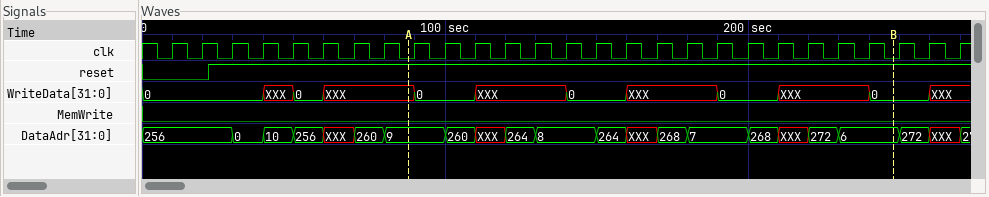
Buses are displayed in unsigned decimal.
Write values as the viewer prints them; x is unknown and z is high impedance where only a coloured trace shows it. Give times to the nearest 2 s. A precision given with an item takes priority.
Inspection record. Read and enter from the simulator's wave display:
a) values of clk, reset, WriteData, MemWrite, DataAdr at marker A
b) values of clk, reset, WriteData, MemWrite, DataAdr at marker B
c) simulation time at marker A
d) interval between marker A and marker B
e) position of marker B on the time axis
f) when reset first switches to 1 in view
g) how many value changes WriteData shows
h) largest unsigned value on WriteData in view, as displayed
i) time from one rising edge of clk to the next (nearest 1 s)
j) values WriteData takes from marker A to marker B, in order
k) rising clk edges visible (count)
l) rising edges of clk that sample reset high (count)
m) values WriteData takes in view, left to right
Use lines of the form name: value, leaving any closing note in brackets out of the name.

values of clk, reset, WriteData, MemWrite, DataAdr at marker A: clk=0, reset=1, WriteData=XXX, MemWrite=0, DataAdr=9
values of clk, reset, WriteData, MemWrite, DataAdr at marker B: clk=0, reset=1, WriteData=0, MemWrite=0, DataAdr=6
simulation time at marker A: 88 s
interval between marker A and marker B: 160 s
position of marker B on the time axis: 248 s
when reset first switches to 1 in view: 22 s
how many value changes WriteData shows: 11
largest unsigned value on WriteData in view, as displayed: 0
time from one rising edge of clk to the next: 10 s
values WriteData takes from marker A to marker B, in order: XXX, 0, XXX, 0, XXX, 0, XXX, 0
rising clk edges visible: 27
rising edges of clk that sample reset high: 25
values WriteData takes in view, left to right: 0, XXX, 0, XXX, 0, XXX, 0, XXX, 0, XXX, 0, XXX
